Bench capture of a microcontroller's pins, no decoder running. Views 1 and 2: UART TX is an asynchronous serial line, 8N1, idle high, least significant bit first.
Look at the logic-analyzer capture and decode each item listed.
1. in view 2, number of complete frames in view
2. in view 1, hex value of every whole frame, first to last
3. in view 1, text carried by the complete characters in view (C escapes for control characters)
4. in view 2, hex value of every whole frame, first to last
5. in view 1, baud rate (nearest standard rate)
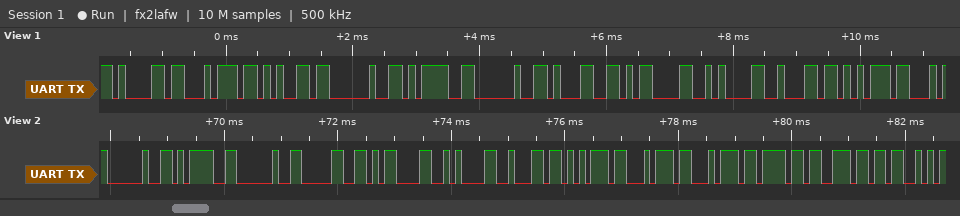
13
61 74 65 20 3D 20 31 0D 0A 62 75
"ate = 1\r\nbu"
20 3D 20 30 0D 0A 62 75 74 74 6F 6E 53
9600 baud
